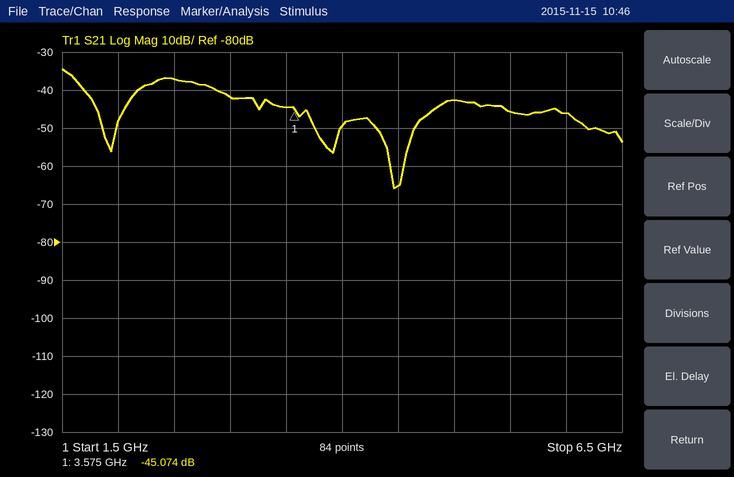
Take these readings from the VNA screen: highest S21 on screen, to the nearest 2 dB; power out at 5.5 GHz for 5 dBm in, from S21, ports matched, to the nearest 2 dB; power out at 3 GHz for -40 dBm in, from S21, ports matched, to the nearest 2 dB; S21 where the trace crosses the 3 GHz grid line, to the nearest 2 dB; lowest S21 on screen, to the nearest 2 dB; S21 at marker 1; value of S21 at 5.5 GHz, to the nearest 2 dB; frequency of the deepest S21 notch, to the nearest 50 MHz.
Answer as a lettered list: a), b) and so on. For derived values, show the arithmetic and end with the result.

a) -34 dB
b) 5 dBm + (-46 dB) = -40 dBm
c) -40 dBm + (-42 dB) = -82 dBm
d) -42 dB
e) -66 dB
f) -45.074 dB
g) -46 dB
h) 4.45 GHz
